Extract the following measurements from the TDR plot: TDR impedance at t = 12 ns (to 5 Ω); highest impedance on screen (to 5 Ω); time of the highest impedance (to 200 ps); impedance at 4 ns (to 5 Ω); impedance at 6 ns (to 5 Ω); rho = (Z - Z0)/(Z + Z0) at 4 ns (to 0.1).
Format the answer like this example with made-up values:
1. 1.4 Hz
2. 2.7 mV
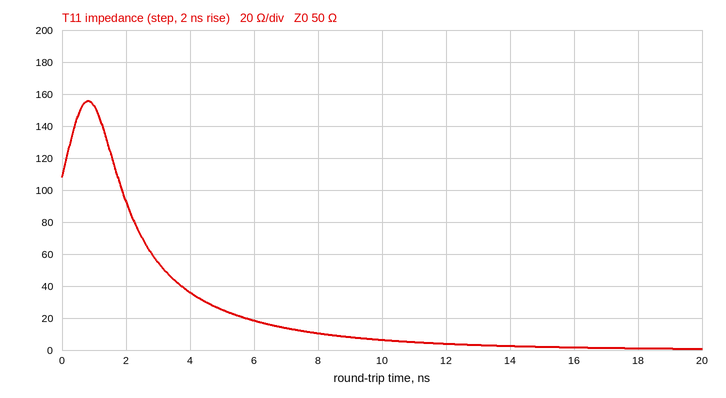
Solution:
1. 5 Ω
2. 155 Ω
3. 800 ps
4. 35 Ω
5. 20 Ω
6. -0.2
